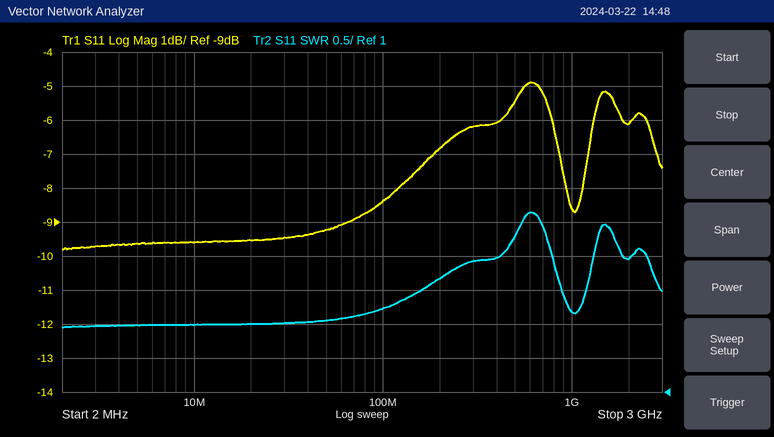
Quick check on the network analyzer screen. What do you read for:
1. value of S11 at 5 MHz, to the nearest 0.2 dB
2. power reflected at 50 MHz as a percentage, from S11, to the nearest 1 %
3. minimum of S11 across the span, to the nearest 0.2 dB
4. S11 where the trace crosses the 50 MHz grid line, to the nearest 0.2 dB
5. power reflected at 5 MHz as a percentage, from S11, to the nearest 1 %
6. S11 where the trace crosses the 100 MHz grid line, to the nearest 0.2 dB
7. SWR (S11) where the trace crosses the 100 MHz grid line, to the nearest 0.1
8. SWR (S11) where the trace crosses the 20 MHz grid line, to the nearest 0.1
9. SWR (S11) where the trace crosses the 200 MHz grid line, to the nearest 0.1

-9.6 dB
12 %
-9.8 dB
-9.2 dB
11 %
-8.4 dB
2.2
2.0
2.7
